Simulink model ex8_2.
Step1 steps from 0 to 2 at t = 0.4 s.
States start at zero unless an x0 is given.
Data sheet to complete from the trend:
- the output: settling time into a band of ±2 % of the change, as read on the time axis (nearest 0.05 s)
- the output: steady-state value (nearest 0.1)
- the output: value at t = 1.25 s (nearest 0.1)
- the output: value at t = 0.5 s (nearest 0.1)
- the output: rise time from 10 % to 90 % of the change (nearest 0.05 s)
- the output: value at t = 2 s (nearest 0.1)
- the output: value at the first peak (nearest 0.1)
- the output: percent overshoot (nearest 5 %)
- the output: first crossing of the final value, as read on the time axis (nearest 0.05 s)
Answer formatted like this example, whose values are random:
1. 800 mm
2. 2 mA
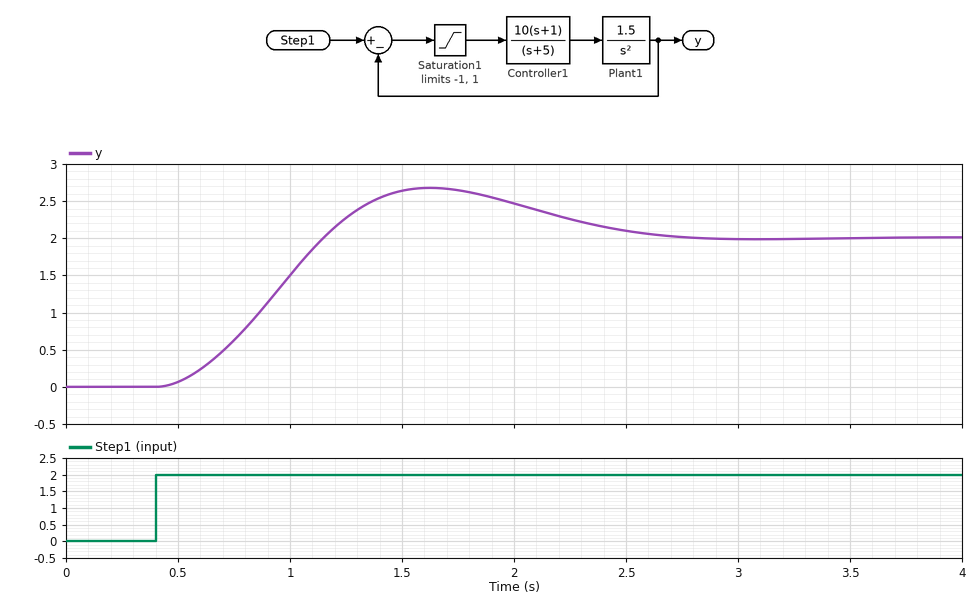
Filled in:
1. 2.65 s
2. 2.0
3. 2.3
4. 0.1
5. 0.50 s
6. 2.5
7. 2.7
8. 35 %
9. 1.15 s
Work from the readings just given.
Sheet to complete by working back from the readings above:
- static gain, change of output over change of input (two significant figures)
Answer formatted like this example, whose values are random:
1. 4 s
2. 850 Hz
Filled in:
1. 1.0
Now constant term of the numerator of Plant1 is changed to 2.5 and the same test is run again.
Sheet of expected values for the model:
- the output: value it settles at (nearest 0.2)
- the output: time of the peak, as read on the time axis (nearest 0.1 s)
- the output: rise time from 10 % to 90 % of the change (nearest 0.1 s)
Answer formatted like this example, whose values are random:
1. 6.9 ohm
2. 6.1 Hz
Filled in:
1. 2.0
2. 1.3 s
3. 0.4 s
